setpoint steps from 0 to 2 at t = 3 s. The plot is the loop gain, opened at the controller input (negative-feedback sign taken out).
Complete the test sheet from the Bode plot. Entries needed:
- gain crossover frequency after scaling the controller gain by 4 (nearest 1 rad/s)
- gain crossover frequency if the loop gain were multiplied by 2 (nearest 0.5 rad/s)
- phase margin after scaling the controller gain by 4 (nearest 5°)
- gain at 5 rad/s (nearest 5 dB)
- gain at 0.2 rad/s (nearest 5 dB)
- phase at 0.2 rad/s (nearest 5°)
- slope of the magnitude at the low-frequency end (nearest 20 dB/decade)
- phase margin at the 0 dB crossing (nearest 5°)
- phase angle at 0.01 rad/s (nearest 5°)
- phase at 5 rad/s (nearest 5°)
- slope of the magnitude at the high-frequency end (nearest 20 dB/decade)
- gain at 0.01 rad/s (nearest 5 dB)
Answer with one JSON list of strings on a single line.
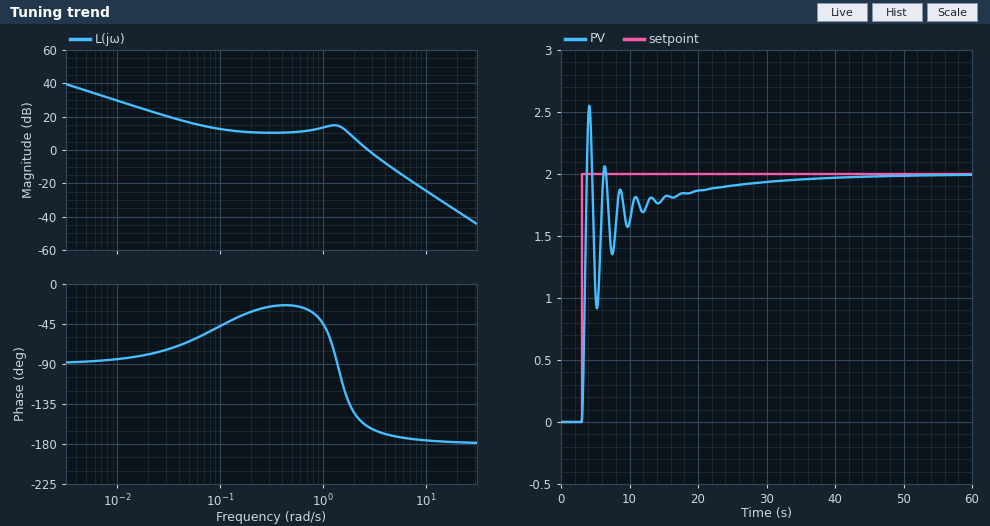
["5 rad/s", "3.5 rad/s", "10°", "-10 dB", "10 dB", "-30°", "-20 dB/decade", "20°", "-85°", "-170°", "-40 dB/decade", "30 dB"]
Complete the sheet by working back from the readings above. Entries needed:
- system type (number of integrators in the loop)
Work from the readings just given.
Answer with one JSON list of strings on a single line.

["1"]
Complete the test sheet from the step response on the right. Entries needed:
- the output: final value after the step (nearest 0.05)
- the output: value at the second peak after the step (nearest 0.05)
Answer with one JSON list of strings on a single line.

["2.00", "2.05"]
